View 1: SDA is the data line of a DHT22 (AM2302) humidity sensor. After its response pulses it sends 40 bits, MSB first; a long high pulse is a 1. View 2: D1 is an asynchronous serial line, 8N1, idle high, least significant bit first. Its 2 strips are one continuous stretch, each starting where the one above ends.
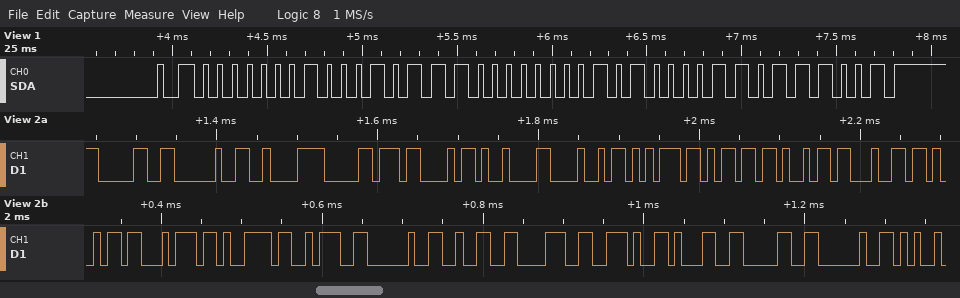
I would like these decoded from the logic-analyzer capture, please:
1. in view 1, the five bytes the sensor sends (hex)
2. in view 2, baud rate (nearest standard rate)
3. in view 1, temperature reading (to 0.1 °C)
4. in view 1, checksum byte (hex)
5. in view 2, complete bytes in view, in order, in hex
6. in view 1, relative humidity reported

01 17 00 A1 B9
115200 baud
16.1 °C
0xB9
30 20 C2 B0 43 09 48 75 6D 69 64 69 74 79 3A 20 32 38 2E 31 30 20
27.9 %
